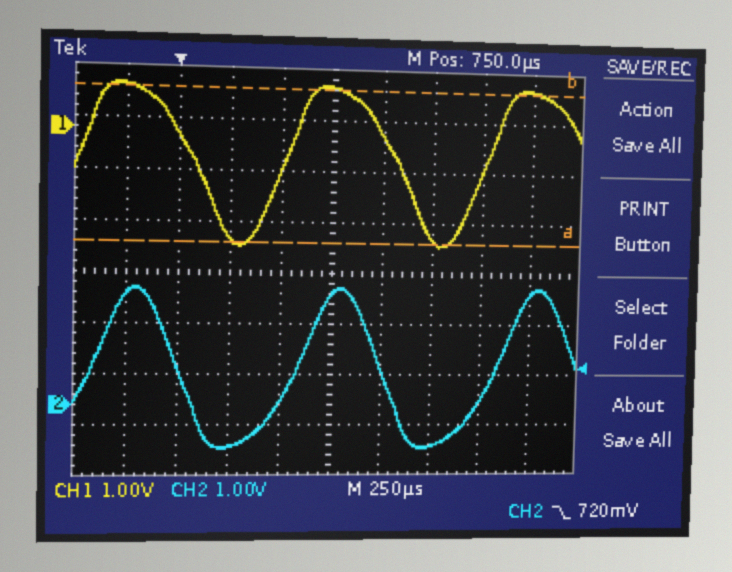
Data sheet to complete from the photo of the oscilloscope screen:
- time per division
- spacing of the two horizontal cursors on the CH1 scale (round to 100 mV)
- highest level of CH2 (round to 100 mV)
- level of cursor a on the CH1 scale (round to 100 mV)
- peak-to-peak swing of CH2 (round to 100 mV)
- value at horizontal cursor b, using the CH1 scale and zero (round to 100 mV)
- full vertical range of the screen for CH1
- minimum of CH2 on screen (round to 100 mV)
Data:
250 µs
3.0 V
2.3 V
-2.2 V
3.2 V
800 mV
8 V
-900 mV
